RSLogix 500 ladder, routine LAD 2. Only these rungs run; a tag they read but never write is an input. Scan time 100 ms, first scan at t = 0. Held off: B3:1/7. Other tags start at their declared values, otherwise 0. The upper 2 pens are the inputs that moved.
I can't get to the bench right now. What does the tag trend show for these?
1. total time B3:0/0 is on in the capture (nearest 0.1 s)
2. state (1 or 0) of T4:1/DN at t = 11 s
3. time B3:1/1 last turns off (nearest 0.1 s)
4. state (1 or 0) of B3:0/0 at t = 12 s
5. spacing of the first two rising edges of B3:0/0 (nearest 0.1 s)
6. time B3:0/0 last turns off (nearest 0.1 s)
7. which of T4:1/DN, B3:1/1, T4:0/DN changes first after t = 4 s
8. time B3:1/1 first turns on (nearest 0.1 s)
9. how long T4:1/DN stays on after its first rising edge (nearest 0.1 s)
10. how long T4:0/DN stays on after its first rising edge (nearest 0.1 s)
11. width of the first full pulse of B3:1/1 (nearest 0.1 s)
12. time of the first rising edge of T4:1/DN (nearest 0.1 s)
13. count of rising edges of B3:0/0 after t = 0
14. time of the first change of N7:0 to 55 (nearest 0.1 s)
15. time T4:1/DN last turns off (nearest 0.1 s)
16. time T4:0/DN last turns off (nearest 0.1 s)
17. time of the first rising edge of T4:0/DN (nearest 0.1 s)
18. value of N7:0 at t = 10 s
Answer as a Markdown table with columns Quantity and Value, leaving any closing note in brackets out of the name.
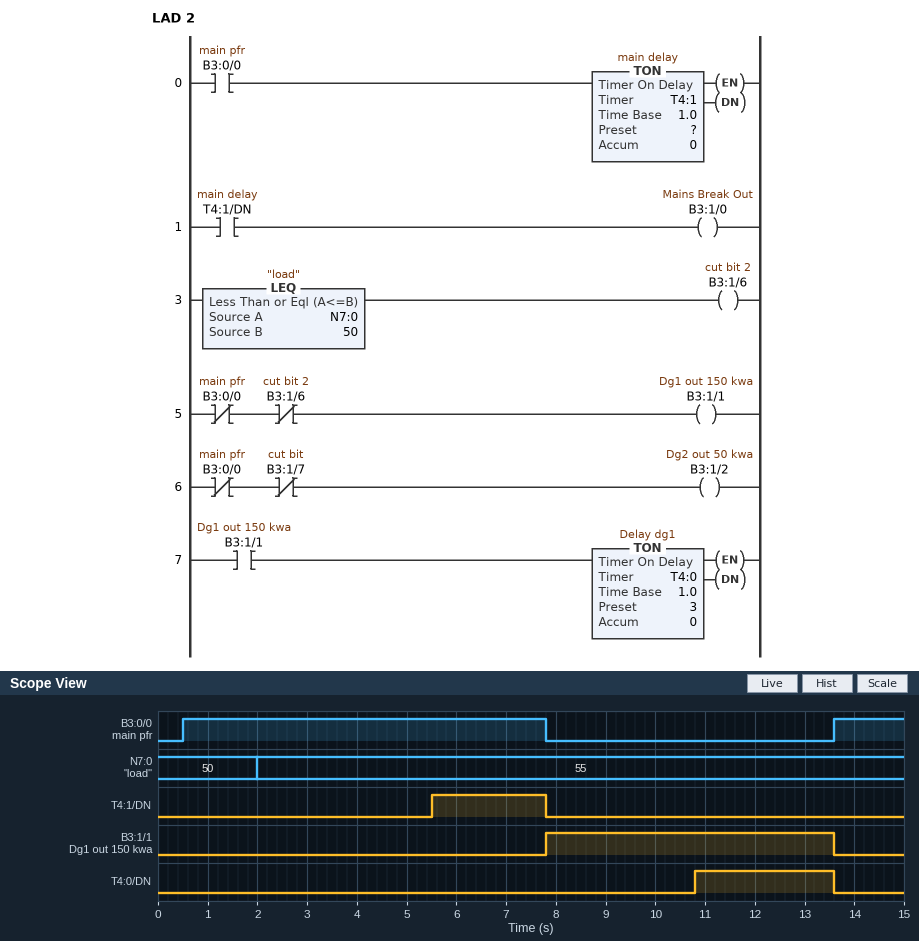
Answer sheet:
| Quantity | Value |
|---|---|
| total time B3:0/0 is on in the capture | 8.7 s |
| state (1 or 0) of T4:1/DN at t = 11 s | 0 |
| time B3:1/1 last turns off | 13.6 s |
| state (1 or 0) of B3:0/0 at t = 12 s | 0 |
| spacing of the first two rising edges of B3:0/0 | 13.1 s |
| time B3:0/0 last turns off | 7.8 s |
| which of T4:1/DN, B3:1/1, T4:0/DN changes first after t = 4 s | T4:1/DN |
| time B3:1/1 first turns on | 7.8 s |
| how long T4:1/DN stays on after its first rising edge | 2.3 s |
| how long T4:0/DN stays on after its first rising edge | 2.8 s |
| width of the first full pulse of B3:1/1 | 5.8 s |
| time of the first rising edge of T4:1/DN | 5.5 s |
| count of rising edges of B3:0/0 after t = 0 | 2 |
| time of the first change of N7:0 to 55 | 2.0 s |
| time T4:1/DN last turns off | 7.8 s |
| time T4:0/DN last turns off | 13.6 s |
| time of the first rising edge of T4:0/DN | 10.8 s |
| value of N7:0 at t = 10 s | 55 |
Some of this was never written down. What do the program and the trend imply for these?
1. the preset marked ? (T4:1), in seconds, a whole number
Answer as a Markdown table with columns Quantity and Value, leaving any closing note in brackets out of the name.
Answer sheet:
| Quantity | Value |
|---|---|
| the preset marked ? (T4:1), in seconds, a whole number | 5 s |
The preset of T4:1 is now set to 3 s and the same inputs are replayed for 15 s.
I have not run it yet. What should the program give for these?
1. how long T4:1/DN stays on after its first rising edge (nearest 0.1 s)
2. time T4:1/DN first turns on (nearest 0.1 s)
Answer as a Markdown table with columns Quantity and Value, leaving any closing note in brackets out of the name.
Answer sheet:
| Quantity | Value |
|---|---|
| how long T4:1/DN stays on after its first rising edge | 4.3 s |
| time T4:1/DN first turns on | 3.5 s |
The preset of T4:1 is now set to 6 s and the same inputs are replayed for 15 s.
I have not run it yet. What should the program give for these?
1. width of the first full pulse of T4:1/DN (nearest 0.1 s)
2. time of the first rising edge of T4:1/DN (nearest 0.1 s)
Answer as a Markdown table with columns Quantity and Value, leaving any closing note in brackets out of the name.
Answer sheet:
| Quantity | Value |
|---|---|
| width of the first full pulse of T4:1/DN | 1.3 s |
| time of the first rising edge of T4:1/DN | 6.5 s |
